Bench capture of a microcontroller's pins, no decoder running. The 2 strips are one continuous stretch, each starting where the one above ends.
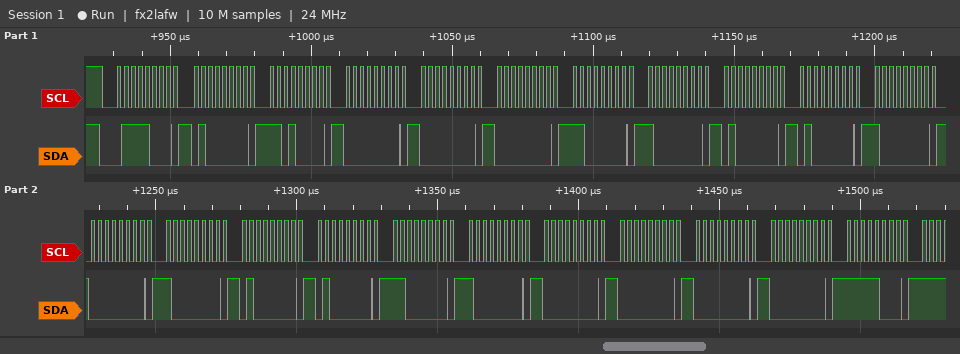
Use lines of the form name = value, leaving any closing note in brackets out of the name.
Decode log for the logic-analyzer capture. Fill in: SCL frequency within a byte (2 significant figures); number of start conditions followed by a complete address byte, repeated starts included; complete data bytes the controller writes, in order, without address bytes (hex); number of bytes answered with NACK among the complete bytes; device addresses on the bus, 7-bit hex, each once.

SCL frequency within a byte = 400 kHz
number of start conditions followed by a complete address byte, repeated starts included = 1
complete data bytes the controller writes, in order, without address bytes = 40 D0 00 00 00 C0 80 40 40 80 00 80 40 40 C0 80 00 00 00 00 F8
number of bytes answered with NACK among the complete bytes = 0
device addresses on the bus, 7-bit hex, each once = 0x3C
